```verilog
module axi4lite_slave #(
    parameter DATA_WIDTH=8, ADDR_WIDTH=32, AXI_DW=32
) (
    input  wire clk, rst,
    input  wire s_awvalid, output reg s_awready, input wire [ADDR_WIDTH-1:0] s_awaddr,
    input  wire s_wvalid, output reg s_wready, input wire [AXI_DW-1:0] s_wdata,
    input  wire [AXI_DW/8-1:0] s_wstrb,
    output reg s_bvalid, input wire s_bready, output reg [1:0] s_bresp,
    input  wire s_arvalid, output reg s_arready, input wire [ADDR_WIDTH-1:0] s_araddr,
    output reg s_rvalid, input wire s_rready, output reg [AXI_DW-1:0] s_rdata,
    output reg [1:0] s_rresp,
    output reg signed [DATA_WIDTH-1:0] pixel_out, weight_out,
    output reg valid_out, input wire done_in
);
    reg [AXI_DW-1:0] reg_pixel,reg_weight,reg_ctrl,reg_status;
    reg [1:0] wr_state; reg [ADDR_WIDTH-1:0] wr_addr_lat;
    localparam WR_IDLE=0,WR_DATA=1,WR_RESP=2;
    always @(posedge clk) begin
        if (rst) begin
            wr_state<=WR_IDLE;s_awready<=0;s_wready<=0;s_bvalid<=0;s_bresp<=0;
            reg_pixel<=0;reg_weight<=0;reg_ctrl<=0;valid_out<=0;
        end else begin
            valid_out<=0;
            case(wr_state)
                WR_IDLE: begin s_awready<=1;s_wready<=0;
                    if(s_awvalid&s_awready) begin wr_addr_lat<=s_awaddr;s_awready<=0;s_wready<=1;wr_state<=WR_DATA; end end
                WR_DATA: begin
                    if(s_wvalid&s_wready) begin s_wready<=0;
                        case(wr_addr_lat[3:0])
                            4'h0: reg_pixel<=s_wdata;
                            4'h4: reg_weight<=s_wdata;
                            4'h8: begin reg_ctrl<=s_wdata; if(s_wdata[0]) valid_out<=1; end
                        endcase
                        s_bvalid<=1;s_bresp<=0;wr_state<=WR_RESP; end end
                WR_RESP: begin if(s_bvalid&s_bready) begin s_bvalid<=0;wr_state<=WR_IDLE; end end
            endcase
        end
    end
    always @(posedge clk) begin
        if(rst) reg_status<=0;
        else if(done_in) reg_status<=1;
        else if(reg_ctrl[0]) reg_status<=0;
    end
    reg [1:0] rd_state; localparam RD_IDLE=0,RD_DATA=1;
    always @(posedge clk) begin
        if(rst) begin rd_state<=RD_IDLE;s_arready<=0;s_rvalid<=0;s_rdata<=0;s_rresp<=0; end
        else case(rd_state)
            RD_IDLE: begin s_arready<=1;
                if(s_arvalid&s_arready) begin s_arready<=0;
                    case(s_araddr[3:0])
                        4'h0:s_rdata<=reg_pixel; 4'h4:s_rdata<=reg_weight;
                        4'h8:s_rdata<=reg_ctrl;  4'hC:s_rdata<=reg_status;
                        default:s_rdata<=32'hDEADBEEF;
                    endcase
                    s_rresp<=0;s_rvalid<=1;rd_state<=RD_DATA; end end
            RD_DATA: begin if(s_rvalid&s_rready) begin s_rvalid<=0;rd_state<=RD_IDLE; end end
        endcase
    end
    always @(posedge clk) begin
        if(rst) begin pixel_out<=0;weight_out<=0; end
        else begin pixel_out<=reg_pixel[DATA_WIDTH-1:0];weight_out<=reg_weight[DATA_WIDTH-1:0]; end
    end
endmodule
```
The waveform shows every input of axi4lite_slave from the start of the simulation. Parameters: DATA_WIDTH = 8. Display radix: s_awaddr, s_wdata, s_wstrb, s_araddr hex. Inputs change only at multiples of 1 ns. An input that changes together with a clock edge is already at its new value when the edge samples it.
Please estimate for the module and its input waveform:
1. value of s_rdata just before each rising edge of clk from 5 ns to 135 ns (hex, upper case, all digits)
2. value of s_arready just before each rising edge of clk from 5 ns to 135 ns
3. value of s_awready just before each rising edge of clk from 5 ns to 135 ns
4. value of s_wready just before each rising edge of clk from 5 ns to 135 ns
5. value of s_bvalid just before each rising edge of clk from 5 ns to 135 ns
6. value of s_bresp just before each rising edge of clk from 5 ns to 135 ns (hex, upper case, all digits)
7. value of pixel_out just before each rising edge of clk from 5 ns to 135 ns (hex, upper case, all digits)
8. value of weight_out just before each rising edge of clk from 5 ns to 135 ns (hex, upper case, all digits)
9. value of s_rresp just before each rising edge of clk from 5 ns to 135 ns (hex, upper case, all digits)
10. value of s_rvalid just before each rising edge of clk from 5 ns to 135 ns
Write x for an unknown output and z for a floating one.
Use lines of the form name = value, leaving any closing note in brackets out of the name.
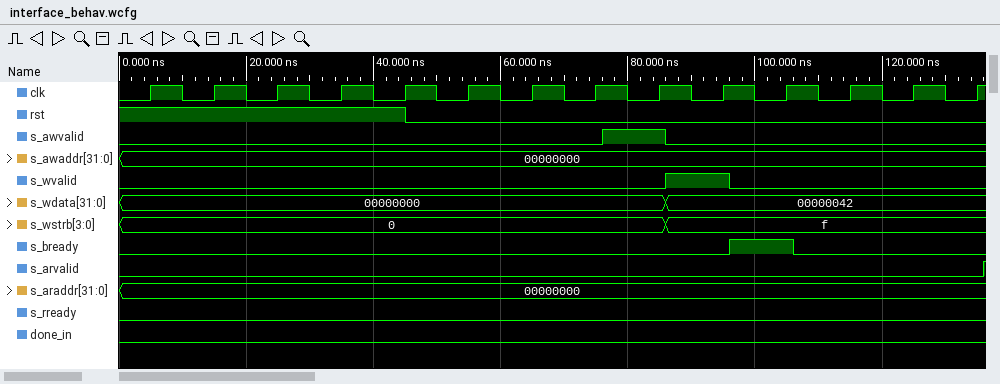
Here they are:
value of s_rdata just before each rising edge of clk from 5 ns to 135 ns = x, 00000000, 00000000, 00000000, 00000000, 00000000, 00000000, 00000000, 00000000, 00000000, 00000000, 00000000, 00000000, 00000000
value of s_arready just before each rising edge of clk from 5 ns to 135 ns = x 0 0 0 0 1 1 1 1 1 1 1 1 1
value of s_awready just before each rising edge of clk from 5 ns to 135 ns = x 0 0 0 0 1 1 1 1 0 0 0 1 1
value of s_wready just before each rising edge of clk from 5 ns to 135 ns = x 0 0 0 0 0 0 0 0 1 0 0 0 0
value of s_bvalid just before each rising edge of clk from 5 ns to 135 ns = x 0 0 0 0 0 0 0 0 0 1 0 0 0
value of s_bresp just before each rising edge of clk from 5 ns to 135 ns = x, 0, 0, 0, 0, 0, 0, 0, 0, 0, 0, 0, 0, 0
value of pixel_out just before each rising edge of clk from 5 ns to 135 ns = x, 00, 00, 00, 00, 00, 00, 00, 00, 00, 00, 42, 42, 42
value of weight_out just before each rising edge of clk from 5 ns to 135 ns = x, 00, 00, 00, 00, 00, 00, 00, 00, 00, 00, 00, 00, 00
value of s_rresp just before each rising edge of clk from 5 ns to 135 ns = x, 0, 0, 0, 0, 0, 0, 0, 0, 0, 0, 0, 0, 0
value of s_rvalid just before each rising edge of clk from 5 ns to 135 ns = x 0 0 0 0 0 0 0 0 0 0 0 0 0
